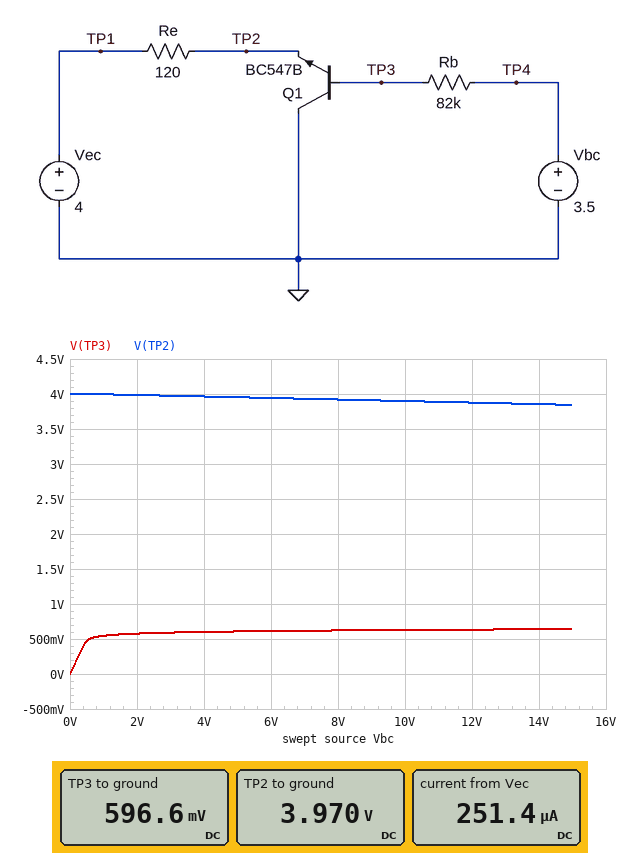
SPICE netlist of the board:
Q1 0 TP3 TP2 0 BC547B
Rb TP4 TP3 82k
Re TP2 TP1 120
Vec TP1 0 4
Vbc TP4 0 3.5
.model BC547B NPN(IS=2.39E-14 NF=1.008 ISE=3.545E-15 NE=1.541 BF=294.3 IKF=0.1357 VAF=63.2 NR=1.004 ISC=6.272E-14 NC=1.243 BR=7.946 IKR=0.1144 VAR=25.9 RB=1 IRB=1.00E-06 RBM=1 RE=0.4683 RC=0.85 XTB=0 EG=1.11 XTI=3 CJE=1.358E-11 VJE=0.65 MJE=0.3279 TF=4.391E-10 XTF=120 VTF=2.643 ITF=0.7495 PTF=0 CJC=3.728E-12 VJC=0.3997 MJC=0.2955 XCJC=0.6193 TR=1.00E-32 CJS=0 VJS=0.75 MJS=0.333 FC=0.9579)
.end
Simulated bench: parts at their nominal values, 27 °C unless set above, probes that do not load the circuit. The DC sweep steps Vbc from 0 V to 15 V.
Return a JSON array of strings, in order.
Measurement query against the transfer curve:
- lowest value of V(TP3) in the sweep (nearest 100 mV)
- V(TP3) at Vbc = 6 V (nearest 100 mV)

["0 V", "600 mV"]
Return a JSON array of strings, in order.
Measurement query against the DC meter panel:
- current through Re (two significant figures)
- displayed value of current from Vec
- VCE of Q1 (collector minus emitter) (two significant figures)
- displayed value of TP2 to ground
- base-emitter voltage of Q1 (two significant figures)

["250 µA", "251.4 µA", "-4.0 V", "3.970 V", "-3.4 V"]
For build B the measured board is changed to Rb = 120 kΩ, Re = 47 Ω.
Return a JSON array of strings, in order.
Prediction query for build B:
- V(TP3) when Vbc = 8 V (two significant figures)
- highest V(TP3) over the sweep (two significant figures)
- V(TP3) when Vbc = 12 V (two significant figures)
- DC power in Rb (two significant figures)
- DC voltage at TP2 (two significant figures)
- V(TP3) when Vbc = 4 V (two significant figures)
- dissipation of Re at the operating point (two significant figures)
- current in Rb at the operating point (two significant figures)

["610 mV", "630 mV", "620 mV", "71 µW", "4.0 V", "590 mV", "1.4 µW", "24 µA"]
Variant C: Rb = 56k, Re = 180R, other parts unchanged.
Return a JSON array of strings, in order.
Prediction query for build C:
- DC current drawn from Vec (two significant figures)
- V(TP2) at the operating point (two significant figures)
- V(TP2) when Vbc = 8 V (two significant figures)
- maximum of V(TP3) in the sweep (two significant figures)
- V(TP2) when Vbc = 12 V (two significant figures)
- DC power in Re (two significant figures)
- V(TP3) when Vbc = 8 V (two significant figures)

["370 µA", "3.9 V", "3.8 V", "650 mV", "3.7 V", "25 µW", "630 mV"]
